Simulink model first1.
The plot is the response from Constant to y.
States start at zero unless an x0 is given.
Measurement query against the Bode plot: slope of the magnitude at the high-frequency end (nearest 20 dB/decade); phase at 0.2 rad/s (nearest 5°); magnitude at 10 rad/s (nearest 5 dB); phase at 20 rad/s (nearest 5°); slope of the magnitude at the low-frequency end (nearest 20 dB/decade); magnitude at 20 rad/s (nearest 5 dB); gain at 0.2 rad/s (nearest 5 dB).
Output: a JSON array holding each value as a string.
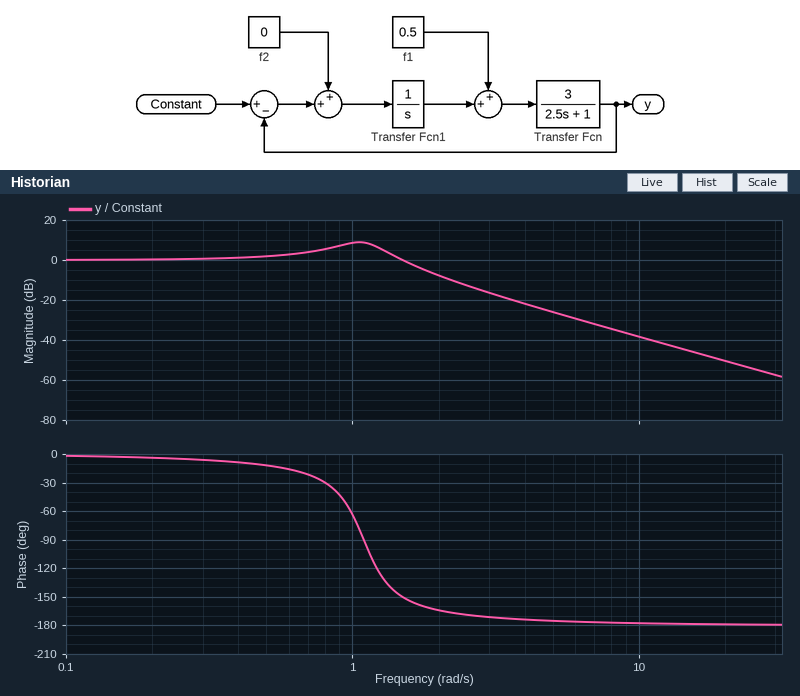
["-40 dB/decade", "-5°", "-40 dB", "-180°", "0 dB/decade", "-50 dB", "0 dB"]
